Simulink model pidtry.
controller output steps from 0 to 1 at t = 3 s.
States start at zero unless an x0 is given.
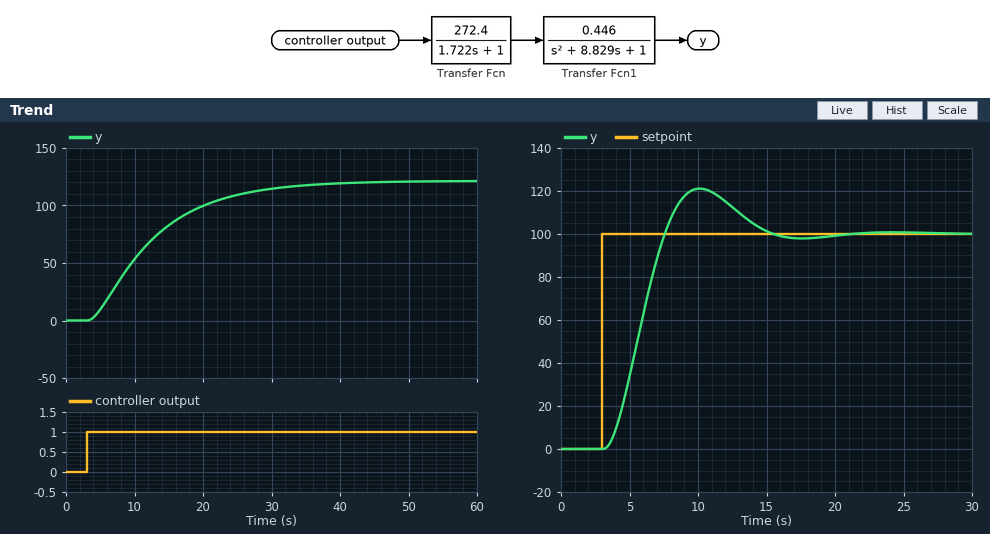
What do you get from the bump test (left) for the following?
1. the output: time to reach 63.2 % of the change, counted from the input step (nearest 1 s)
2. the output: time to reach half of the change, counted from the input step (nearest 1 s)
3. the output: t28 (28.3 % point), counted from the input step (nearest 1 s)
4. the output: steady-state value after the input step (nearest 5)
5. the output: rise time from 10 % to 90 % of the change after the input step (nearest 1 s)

11 s
8 s
5 s
120
20 s
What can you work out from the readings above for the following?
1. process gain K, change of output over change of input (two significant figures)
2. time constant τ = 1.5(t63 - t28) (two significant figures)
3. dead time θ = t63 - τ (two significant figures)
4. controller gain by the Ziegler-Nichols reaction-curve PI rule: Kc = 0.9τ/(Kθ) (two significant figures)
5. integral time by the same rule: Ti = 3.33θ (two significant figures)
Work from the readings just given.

120
9.0 s
2.0 s
0.034
6.7 s
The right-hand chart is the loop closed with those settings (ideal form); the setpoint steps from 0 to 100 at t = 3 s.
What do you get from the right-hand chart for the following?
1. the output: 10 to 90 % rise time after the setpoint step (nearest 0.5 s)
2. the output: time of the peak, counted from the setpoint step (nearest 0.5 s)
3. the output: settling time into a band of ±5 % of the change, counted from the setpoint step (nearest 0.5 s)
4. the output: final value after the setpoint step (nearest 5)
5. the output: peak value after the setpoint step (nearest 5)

3.0 s
7.0 s
11.0 s
100
120
